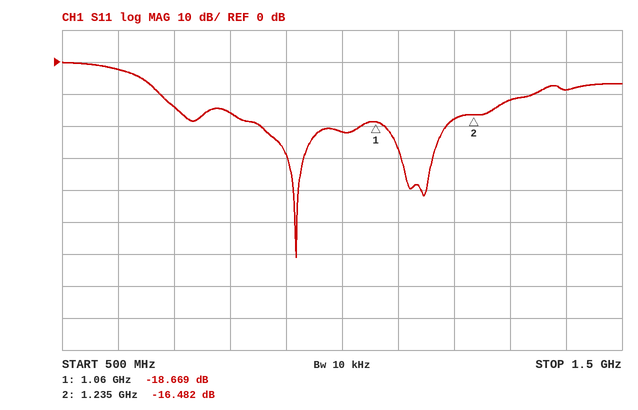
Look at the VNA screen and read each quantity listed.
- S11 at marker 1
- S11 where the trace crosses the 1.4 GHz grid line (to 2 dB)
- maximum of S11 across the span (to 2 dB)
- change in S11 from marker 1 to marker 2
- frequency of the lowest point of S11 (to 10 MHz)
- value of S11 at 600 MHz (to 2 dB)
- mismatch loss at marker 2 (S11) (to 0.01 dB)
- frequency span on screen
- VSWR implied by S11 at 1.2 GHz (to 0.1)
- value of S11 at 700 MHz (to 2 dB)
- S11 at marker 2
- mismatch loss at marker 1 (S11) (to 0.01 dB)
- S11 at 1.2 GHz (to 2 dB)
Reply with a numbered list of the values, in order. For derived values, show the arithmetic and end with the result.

1. -18.669 dB
2. -8 dB
3. 0 dB
4. -16.482 − (-18.669) = 2.187 dB
5. 920 MHz
6. -2 dB
7. −10 log10(1 − 10^(-16.482/10)) ≈ 0.10 dB
8. 1 GHz
9. |Γ| = 10^(-18/20) = 0.1259; VSWR = (1 + 0.1259)/(1 − 0.1259) ≈ 1.3
10. -14 dB
11. -16.482 dB
12. −10 log10(1 − 10^(-18.669/10)) ≈ 0.06 dB
13. -18 dB
